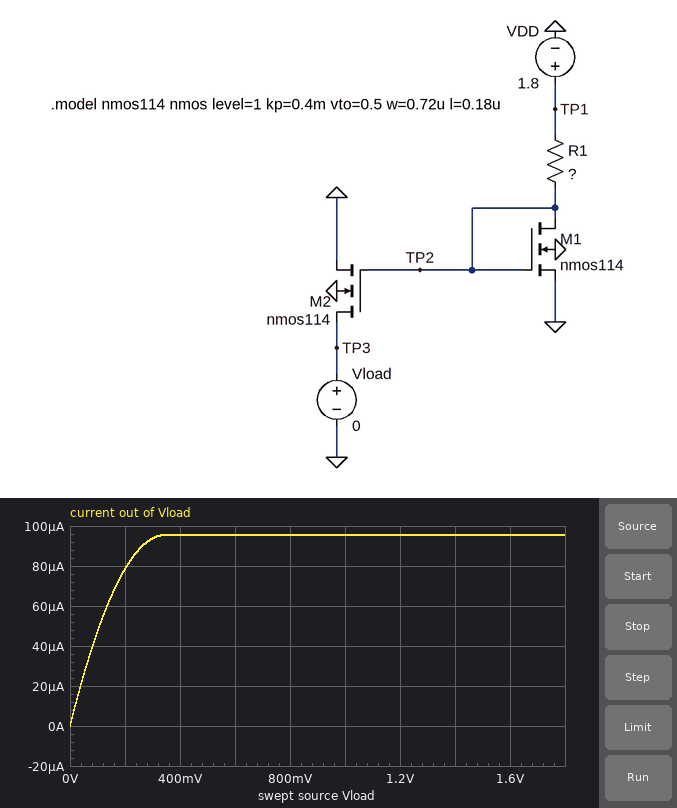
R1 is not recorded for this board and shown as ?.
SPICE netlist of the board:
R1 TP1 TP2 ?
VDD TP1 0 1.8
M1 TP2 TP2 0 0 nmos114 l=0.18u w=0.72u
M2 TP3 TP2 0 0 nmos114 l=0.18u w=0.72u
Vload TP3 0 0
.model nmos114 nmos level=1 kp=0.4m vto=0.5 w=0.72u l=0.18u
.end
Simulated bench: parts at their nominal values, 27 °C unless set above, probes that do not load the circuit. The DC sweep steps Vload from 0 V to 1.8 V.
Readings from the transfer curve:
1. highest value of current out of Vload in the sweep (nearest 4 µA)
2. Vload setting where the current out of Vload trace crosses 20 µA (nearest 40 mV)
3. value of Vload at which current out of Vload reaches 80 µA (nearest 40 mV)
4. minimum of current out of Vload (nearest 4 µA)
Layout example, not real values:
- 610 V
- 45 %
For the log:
- 96 µA
- 40 mV
- 200 mV
- 0 A
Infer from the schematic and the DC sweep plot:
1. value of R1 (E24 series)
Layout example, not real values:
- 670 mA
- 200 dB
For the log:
- 10 kΩ
